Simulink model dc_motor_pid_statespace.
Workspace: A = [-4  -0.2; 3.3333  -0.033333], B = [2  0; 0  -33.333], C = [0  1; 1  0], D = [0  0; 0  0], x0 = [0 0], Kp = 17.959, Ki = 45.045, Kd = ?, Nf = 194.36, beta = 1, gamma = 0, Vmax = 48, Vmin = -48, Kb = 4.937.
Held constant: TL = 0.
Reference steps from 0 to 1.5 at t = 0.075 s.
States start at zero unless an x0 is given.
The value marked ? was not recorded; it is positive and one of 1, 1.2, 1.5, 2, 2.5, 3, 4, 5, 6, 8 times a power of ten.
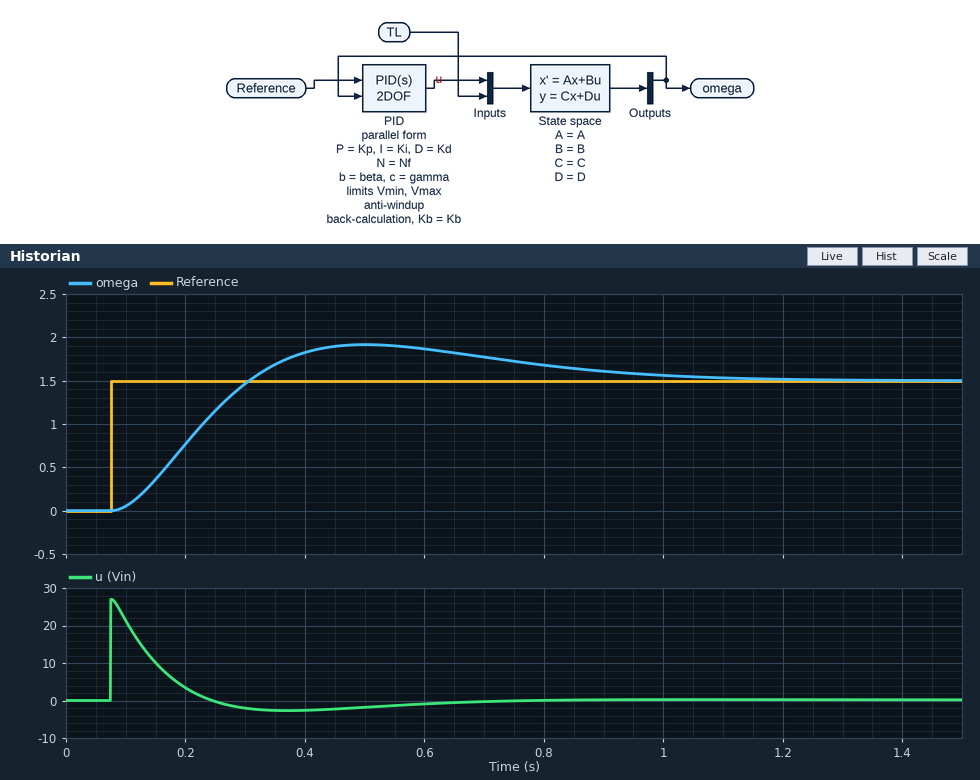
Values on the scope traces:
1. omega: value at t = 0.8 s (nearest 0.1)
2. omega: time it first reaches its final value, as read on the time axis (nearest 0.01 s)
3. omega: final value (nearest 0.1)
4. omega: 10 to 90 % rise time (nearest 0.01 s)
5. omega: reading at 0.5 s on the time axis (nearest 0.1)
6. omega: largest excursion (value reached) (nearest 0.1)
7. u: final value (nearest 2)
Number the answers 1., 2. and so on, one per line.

1. 1.7
2. 0.31 s
3. 1.5
4. 0.16 s
5. 1.9
6. 1.9
7. 0
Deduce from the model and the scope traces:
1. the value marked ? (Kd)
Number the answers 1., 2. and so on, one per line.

1. 2
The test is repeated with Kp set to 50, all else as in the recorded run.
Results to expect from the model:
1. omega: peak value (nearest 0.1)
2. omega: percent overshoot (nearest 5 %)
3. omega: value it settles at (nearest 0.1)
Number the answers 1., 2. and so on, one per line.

1. 1.8
2. 20 %
3. 1.5
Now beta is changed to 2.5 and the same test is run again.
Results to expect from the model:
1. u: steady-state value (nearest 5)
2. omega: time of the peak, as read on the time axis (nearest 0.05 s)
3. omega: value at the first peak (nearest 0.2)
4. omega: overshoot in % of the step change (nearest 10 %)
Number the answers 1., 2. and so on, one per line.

1. 0
2. 0.40 s
3. 3.6
4. 140 %
